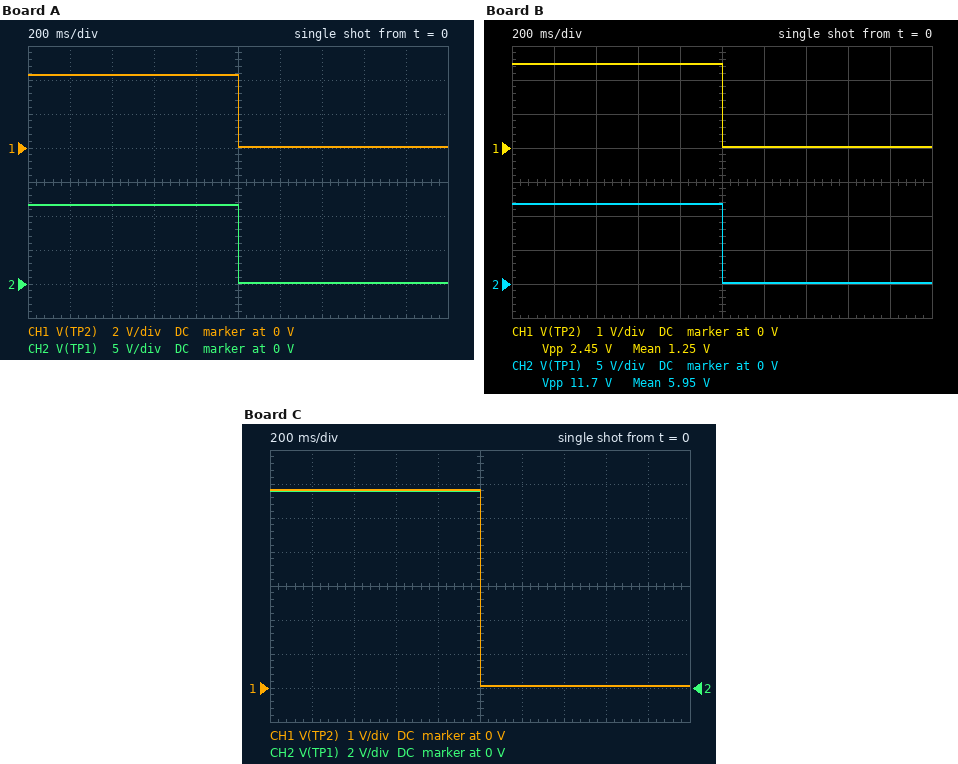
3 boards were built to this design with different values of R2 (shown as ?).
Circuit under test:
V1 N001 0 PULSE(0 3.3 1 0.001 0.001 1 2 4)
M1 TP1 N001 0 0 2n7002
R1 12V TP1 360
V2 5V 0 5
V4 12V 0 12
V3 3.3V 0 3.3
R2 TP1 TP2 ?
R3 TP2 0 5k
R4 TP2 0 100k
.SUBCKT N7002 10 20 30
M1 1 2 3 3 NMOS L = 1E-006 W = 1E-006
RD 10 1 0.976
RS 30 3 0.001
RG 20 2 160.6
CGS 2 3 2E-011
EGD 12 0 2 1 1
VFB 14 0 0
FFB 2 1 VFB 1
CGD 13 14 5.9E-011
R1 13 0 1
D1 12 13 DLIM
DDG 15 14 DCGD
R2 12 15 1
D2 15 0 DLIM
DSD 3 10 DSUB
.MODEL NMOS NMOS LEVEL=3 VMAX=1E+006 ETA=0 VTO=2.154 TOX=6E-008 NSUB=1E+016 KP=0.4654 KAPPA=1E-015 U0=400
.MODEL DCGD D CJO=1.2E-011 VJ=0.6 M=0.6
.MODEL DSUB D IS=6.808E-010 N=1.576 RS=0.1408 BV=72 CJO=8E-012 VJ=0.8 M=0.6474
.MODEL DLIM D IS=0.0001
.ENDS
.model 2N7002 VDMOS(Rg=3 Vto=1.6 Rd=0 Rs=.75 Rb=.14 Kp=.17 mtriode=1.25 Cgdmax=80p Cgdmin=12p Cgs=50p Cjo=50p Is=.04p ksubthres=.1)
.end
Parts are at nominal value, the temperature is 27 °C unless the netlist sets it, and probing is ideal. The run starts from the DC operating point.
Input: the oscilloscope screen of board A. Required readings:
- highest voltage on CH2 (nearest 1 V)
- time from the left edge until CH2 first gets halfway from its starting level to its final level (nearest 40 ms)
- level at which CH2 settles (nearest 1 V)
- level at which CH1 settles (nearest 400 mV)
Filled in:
12 V
1.00 s
0 V
0 V
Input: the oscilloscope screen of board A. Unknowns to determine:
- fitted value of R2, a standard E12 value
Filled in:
8.2 kΩ
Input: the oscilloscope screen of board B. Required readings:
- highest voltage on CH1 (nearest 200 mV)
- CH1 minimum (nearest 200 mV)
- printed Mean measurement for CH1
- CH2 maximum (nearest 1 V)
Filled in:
2.4 V
0 V
1.25 V
12 V
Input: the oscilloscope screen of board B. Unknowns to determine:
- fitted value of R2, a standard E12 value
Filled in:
18 kΩ
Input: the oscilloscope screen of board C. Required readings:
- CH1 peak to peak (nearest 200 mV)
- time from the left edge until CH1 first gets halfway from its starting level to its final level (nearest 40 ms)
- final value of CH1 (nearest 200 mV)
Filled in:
5.8 V
1.00 s
0 V
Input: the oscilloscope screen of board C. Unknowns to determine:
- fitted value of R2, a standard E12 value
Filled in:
4.7 kΩ
